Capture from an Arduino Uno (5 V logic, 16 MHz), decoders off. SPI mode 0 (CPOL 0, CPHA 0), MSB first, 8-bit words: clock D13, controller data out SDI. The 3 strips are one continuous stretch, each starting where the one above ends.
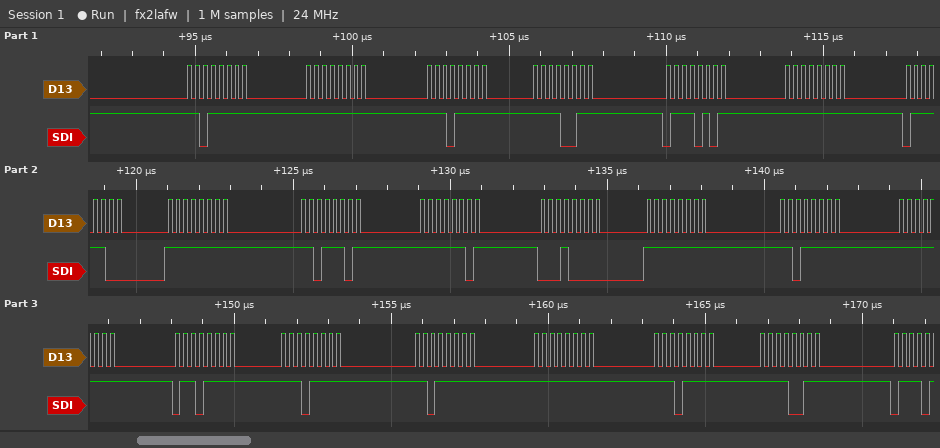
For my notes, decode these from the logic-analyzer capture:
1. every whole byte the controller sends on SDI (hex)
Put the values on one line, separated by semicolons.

DF FF EF F3 75 FF 7C FF DD FD 10 FF DF FF 6F EF DF FF EF F3
